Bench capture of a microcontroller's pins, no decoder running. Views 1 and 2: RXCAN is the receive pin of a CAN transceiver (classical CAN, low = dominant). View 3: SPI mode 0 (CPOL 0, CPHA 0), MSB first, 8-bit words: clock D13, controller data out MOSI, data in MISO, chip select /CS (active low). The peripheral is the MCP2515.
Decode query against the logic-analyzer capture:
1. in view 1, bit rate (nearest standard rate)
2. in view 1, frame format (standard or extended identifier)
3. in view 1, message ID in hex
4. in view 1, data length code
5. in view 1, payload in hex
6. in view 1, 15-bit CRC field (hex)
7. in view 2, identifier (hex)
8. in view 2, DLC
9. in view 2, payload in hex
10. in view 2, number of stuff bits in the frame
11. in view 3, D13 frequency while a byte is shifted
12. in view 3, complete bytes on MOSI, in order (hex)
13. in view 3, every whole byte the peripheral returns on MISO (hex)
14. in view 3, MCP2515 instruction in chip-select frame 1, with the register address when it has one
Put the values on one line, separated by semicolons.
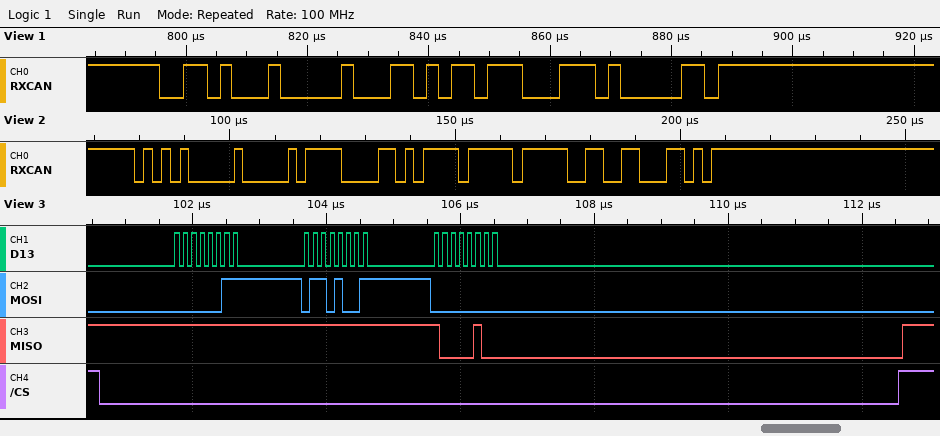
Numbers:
500 kbit/s; standard; 0x344; 1; AD; 0x63A0; 0x540; 3; C3 5E FF; 4; 8 MHz; 03 69 00; FF FF 84; READ 0x69
